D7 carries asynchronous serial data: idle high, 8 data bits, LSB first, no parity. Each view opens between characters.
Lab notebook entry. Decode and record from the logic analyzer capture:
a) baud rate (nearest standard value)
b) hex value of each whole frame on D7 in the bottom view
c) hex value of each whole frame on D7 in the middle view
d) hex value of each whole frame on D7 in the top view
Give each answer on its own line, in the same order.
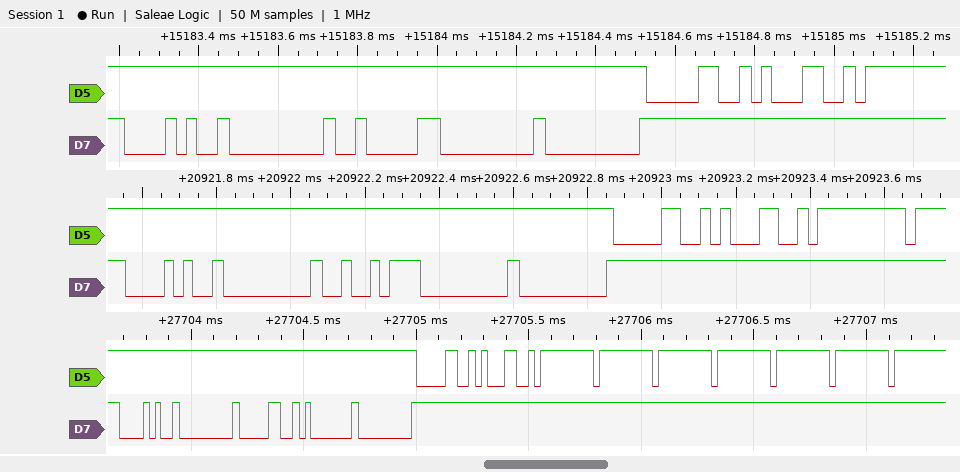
38400 baud
28, 00, 30, 01, 00
28, 00, D2, 00, 00
28, 00, 82, 00, 00
